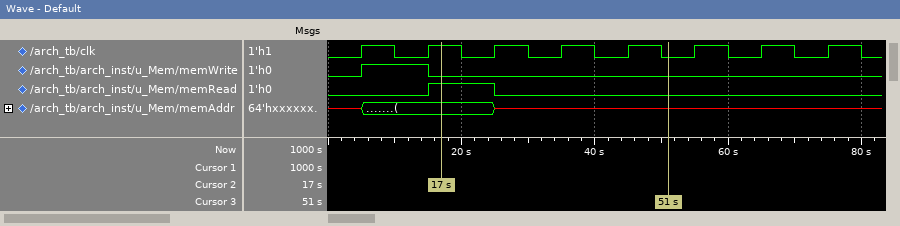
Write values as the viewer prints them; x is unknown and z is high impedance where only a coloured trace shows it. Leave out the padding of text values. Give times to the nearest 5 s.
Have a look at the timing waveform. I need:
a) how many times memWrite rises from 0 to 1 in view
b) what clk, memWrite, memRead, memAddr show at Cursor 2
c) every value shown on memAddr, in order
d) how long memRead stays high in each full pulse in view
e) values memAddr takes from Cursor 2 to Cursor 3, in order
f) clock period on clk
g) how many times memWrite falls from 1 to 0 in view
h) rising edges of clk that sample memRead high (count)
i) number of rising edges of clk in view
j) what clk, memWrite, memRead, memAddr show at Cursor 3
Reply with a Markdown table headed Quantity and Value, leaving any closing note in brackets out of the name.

| Quantity | Value |
|---|---|
| how many times memWrite rises from 0 to 1 in view | 1 |
| what clk, memWrite, memRead, memAddr show at Cursor 2 | clk=1, memWrite=0, memRead=1, memAddr=( |
| every value shown on memAddr, in order | x, (, x |
| how long memRead stays high in each full pulse in view | 10 s |
| values memAddr takes from Cursor 2 to Cursor 3, in order | (, x |
| clock period on clk | 10 s |
| how many times memWrite falls from 1 to 0 in view | 1 |
| rising edges of clk that sample memRead high | 1 |
| number of rising edges of clk in view | 8 |
| what clk, memWrite, memRead, memAddr show at Cursor 3 | clk=0, memWrite=0, memRead=0, memAddr=x |
